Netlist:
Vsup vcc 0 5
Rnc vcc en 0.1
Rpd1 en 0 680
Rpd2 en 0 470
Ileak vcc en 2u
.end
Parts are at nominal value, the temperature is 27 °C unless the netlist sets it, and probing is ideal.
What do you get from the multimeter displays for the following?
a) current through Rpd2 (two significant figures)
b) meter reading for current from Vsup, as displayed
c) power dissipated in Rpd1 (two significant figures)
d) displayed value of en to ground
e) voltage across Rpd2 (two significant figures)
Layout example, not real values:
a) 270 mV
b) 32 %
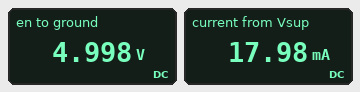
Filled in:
a) 11 mA
b) 17.98 mA
c) 37 mW
d) 4.998 V
e) 5.0 V
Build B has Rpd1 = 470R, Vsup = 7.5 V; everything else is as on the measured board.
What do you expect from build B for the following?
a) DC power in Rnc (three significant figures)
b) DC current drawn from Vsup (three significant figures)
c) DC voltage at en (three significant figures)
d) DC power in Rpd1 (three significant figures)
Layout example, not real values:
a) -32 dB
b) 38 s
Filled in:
a) 102 µW
b) 31.9 mA
c) 7.50 V
d) 120 mW
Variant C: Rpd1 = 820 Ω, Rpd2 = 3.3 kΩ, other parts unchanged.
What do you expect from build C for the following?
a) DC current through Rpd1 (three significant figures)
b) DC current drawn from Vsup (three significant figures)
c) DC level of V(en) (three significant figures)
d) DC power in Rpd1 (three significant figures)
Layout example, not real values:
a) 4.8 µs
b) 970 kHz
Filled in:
a) 6.10 mA
b) 7.61 mA
c) 5.00 V
d) 30.5 mW
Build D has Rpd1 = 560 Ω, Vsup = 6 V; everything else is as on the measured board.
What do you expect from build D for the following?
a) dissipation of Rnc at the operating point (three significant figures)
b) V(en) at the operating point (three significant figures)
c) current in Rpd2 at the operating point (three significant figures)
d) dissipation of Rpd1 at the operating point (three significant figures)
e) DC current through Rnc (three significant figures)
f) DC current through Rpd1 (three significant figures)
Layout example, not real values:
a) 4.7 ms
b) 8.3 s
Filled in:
a) 55.1 µW
b) 6.00 V
c) 12.8 mA
d) 64.2 mW
e) 23.5 mA
f) 10.7 mA
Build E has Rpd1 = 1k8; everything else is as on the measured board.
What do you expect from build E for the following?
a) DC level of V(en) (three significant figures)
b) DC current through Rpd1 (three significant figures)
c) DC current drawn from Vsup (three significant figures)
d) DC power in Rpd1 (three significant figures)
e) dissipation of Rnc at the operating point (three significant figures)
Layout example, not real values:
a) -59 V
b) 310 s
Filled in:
a) 5.00 V
b) 2.78 mA
c) 13.4 mA
d) 13.9 mW
e) 18.0 µW
